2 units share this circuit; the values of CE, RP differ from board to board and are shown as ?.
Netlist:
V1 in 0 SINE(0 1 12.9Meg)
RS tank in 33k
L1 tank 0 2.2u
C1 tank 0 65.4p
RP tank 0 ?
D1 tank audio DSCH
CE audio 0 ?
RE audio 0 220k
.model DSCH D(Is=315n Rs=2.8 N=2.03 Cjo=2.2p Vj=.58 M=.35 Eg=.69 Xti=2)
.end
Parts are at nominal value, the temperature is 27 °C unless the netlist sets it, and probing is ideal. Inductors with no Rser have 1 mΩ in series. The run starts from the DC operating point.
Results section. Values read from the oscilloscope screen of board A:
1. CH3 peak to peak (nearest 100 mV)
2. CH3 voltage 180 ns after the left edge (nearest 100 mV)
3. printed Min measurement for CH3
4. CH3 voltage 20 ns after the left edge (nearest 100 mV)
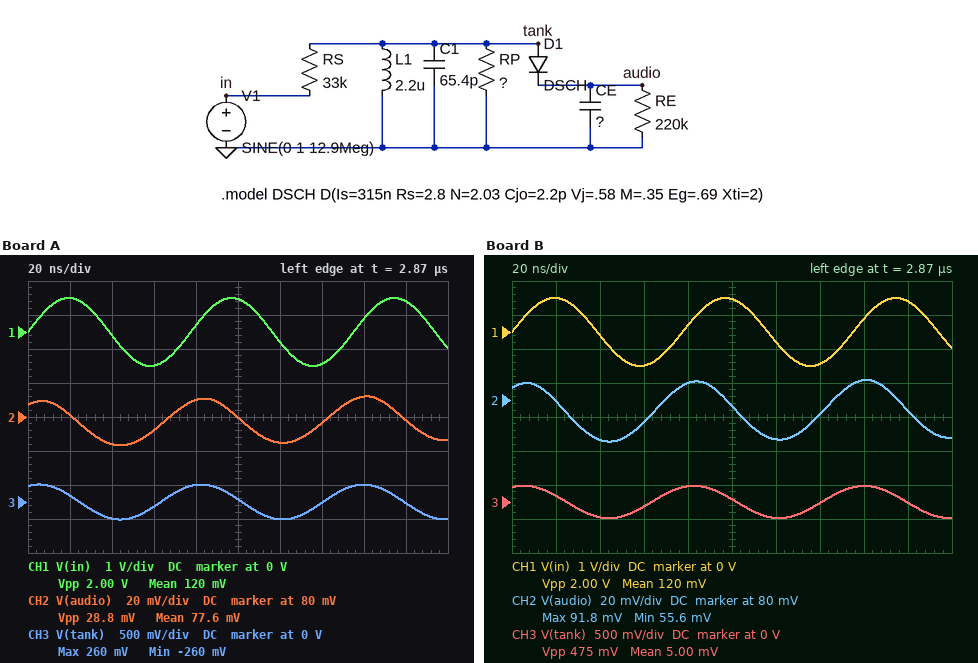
500 mV
0 V
-260 mV
100 mV
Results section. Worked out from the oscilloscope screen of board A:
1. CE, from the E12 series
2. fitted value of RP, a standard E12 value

39 pF
68 kΩ
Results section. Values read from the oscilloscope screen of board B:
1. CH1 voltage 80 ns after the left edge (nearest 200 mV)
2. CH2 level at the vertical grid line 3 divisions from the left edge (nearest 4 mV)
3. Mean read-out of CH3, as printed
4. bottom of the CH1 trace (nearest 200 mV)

200 mV
68 mV
5.00 mV
-1.0 V
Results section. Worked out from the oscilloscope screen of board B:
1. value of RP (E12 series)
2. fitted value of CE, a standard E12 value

39 kΩ
27 pF
